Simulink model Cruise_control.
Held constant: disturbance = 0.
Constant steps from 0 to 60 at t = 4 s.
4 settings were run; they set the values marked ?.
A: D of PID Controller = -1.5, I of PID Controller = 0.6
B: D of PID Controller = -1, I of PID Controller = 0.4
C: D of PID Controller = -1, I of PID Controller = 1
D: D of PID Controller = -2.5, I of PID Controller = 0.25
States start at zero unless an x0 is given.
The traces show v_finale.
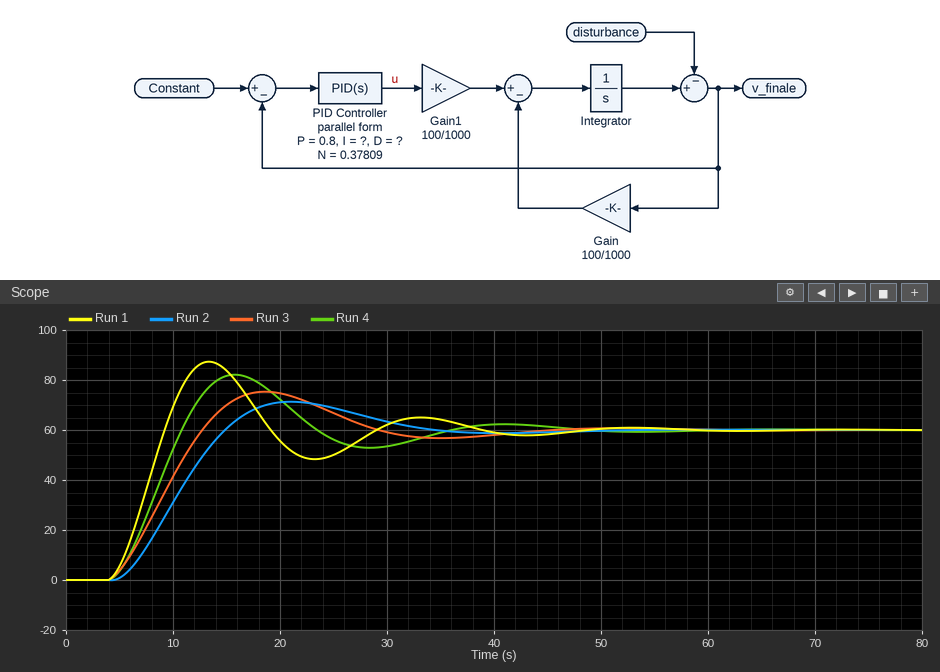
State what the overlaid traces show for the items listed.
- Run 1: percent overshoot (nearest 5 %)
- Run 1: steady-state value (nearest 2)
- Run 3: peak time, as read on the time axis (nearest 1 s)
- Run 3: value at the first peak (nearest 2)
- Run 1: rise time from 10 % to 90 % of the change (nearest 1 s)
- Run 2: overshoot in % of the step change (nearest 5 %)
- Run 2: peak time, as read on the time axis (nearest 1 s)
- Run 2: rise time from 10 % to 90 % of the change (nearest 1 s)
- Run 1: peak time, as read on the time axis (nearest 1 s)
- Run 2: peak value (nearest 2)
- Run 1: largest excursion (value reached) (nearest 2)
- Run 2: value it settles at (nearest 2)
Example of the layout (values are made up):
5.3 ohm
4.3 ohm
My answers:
45 %
60
19 s
76
4 s
20 %
21 s
7 s
13 s
72
88
60
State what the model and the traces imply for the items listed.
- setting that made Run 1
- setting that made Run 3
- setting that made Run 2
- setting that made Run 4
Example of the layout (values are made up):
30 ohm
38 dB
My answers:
C
B
D
A
